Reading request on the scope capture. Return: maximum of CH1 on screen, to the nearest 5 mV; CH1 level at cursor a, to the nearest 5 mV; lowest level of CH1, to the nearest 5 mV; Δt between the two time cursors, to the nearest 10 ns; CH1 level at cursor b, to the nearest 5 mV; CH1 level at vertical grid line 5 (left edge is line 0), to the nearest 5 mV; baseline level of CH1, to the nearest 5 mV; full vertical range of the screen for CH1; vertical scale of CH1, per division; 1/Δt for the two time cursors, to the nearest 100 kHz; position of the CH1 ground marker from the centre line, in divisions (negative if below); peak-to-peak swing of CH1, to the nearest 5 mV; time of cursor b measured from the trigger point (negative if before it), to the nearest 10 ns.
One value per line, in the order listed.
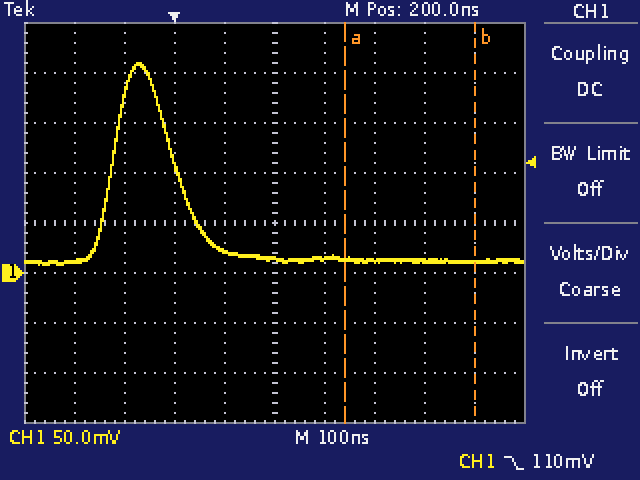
210 mV
15 mV
10 mV
260 ns
10 mV
15 mV
10 mV
400 mV
50 mV
3.8 MHz
-1.0 div
200 mV
+600 ns
